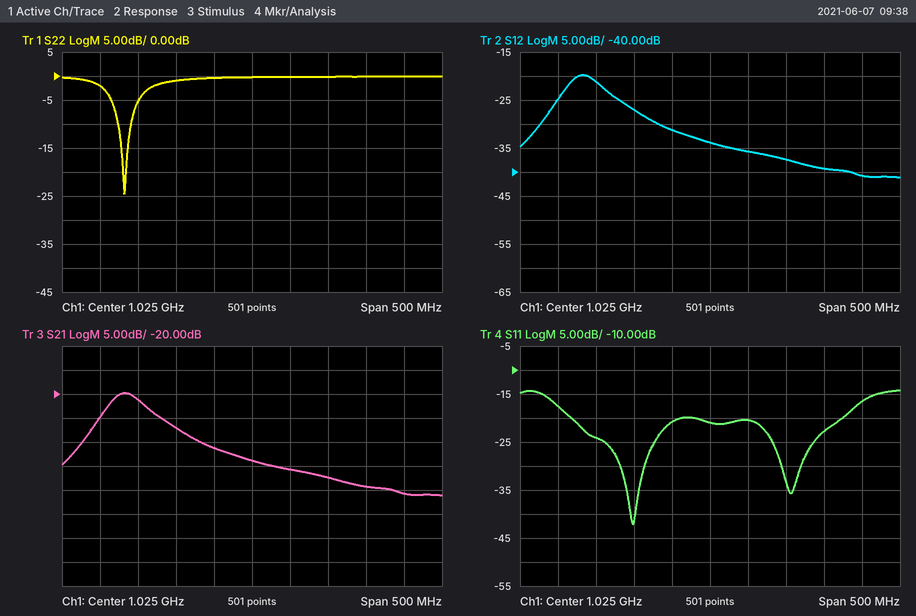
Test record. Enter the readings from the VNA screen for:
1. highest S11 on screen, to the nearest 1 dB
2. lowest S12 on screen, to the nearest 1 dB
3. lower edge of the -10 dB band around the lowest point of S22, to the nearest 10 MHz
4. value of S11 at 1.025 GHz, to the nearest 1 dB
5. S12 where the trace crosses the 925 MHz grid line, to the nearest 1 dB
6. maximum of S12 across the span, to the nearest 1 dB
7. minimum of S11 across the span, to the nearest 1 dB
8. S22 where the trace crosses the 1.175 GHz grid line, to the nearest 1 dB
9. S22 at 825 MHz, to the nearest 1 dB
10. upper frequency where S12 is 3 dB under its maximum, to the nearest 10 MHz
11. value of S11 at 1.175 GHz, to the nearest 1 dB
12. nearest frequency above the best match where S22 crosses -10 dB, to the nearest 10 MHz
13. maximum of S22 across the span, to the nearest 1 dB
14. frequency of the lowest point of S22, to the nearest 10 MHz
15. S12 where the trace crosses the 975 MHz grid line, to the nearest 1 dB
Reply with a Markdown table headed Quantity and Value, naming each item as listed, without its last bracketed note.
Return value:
| Quantity | Value |
|---|---|
| highest S11 on screen, to the nearest 1 dB | -14 dB |
| lowest S12 on screen, to the nearest 1 dB | -41 dB |
| lower edge of the -10 dB band around the lowest point of S22, to the nearest 10 MHz | 850 MHz |
| value of S11 at 1.025 GHz, to the nearest 1 dB | -21 dB |
| S12 where the trace crosses the 925 MHz grid line, to the nearest 1 dB | -27 dB |
| maximum of S12 across the span, to the nearest 1 dB | -20 dB |
| minimum of S11 across the span, to the nearest 1 dB | -42 dB |
| S22 where the trace crosses the 1.175 GHz grid line, to the nearest 1 dB | 0 dB |
| S22 at 825 MHz, to the nearest 1 dB | -2 dB |
| upper frequency where S12 is 3 dB under its maximum, to the nearest 10 MHz | 890 MHz |
| value of S11 at 1.175 GHz, to the nearest 1 dB | -23 dB |
| nearest frequency above the best match where S22 crosses -10 dB, to the nearest 10 MHz | 870 MHz |
| maximum of S22 across the span, to the nearest 1 dB | 0 dB |
| frequency of the lowest point of S22, to the nearest 10 MHz | 860 MHz |
| S12 where the trace crosses the 975 MHz grid line, to the nearest 1 dB | -31 dB |
